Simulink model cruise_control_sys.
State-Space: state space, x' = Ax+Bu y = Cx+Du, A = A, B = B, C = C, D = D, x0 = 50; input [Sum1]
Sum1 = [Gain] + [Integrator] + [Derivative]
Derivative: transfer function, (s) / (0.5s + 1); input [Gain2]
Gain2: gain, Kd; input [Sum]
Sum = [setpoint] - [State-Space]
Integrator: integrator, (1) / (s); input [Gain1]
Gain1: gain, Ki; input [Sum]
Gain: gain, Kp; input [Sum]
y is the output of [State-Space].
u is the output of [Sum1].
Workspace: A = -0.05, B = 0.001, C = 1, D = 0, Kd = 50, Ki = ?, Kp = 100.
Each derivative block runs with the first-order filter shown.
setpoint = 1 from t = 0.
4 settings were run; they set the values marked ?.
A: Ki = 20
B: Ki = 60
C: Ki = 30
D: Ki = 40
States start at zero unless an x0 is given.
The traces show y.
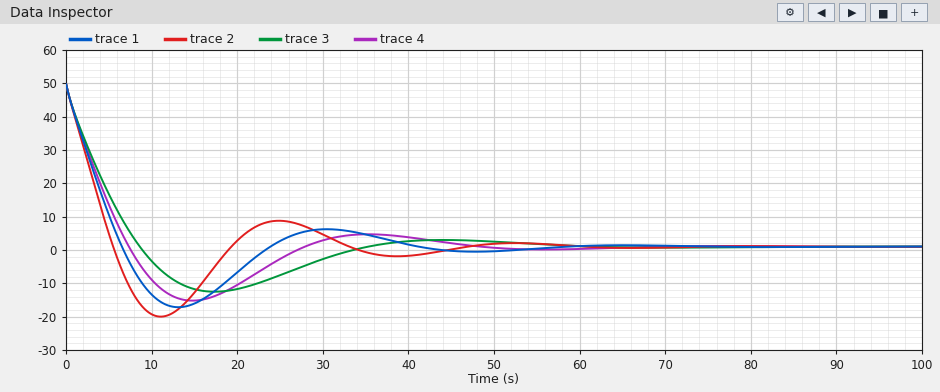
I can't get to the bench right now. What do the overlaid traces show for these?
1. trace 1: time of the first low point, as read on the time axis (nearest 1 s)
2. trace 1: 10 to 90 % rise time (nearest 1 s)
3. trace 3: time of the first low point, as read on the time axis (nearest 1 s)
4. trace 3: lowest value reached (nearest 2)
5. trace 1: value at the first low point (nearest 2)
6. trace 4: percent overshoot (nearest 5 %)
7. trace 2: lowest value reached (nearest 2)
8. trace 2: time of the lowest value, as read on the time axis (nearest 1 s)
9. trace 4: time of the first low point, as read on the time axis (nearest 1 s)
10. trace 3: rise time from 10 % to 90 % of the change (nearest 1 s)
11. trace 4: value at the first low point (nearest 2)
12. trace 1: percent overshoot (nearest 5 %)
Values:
13 s
5 s
17 s
-12
-18
35 %
-20
11 s
15 s
7 s
-16
35 %
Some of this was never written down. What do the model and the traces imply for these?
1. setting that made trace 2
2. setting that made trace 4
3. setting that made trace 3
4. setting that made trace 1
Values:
B
C
A
D
